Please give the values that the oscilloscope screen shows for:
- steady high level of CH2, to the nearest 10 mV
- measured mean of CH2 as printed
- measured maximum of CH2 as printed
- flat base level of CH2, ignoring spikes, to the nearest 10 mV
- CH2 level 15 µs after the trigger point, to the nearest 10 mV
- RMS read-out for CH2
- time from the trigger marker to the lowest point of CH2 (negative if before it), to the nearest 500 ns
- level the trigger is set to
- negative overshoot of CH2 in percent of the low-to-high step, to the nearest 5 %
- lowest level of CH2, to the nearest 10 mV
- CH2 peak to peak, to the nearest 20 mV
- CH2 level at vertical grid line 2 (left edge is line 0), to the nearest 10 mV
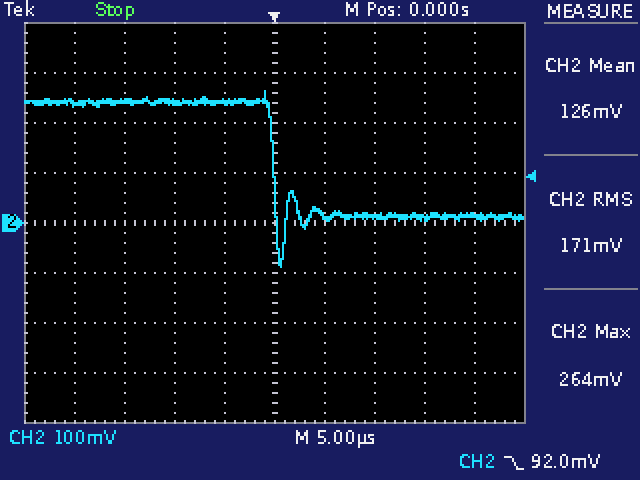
240 mV
126 mV
264 mV
10 mV
10 mV
171 mV
+500 ns
92.0 mV
45 %
-90 mV
360 mV
240 mV
